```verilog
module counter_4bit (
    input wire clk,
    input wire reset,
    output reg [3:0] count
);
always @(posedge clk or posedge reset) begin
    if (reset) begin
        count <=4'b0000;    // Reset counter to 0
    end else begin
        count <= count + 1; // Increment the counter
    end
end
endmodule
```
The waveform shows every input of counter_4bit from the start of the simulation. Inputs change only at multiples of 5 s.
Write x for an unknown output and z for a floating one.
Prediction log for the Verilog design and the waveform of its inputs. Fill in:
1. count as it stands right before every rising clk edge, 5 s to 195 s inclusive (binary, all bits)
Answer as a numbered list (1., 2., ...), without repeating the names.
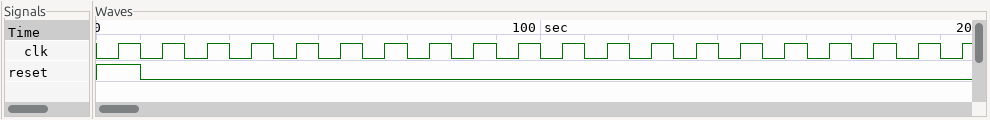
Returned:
1. 0000, 0000, 0001, 0010, 0011, 0100, 0101, 0110, 0111, 1000, 1001, 1010, 1011, 1100, 1101, 1110, 1111, 0000, 0001, 0010
